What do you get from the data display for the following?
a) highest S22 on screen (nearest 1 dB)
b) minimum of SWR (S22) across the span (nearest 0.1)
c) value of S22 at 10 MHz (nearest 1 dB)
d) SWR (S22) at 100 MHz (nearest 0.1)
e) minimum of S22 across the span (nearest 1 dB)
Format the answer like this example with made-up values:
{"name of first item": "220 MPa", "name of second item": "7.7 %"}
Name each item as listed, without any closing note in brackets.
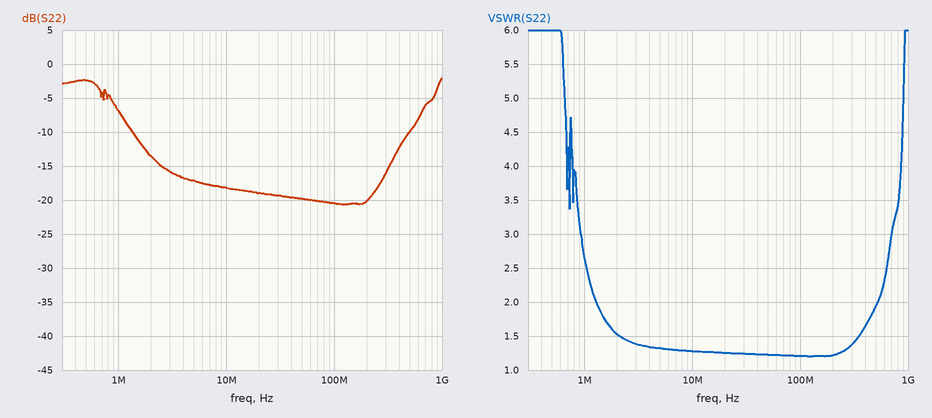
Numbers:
{"highest S22 on screen": "-2 dB", "minimum of SWR (S22) across the span": "1.2", "value of S22 at 10 MHz": "-18 dB", "SWR (S22) at 100 MHz": "1.2", "minimum of S22 across the span": "-21 dB"}
